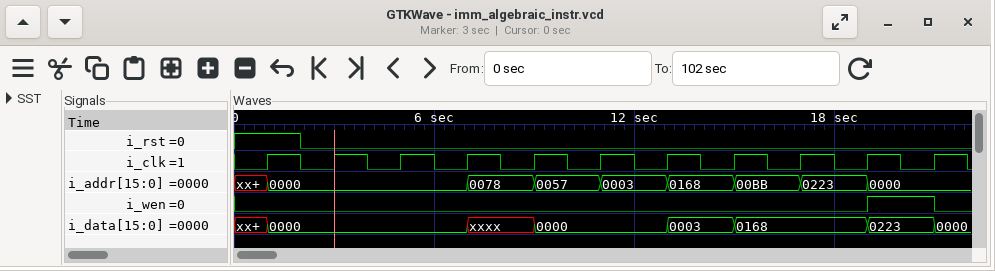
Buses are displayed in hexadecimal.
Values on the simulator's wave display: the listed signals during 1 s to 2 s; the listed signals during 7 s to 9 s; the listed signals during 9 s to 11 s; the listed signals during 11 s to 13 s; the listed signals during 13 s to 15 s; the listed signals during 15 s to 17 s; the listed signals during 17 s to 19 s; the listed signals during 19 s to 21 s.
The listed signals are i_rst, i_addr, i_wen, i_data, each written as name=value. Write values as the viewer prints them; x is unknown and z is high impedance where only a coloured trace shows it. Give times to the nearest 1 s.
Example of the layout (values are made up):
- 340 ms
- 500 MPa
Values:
- i_rst=1, i_addr=0000, i_wen=0, i_data=0000
- i_rst=0, i_addr=0078, i_wen=0, i_data=xxxx
- i_rst=0, i_addr=0057, i_wen=0, i_data=0000
- i_rst=0, i_addr=0003, i_wen=0, i_data=0000
- i_rst=0, i_addr=0168, i_wen=0, i_data=0003
- i_rst=0, i_addr=00BB, i_wen=0, i_data=0168
- i_rst=0, i_addr=0223, i_wen=0, i_data=0168
- i_rst=0, i_addr=0000, i_wen=1, i_data=0223
